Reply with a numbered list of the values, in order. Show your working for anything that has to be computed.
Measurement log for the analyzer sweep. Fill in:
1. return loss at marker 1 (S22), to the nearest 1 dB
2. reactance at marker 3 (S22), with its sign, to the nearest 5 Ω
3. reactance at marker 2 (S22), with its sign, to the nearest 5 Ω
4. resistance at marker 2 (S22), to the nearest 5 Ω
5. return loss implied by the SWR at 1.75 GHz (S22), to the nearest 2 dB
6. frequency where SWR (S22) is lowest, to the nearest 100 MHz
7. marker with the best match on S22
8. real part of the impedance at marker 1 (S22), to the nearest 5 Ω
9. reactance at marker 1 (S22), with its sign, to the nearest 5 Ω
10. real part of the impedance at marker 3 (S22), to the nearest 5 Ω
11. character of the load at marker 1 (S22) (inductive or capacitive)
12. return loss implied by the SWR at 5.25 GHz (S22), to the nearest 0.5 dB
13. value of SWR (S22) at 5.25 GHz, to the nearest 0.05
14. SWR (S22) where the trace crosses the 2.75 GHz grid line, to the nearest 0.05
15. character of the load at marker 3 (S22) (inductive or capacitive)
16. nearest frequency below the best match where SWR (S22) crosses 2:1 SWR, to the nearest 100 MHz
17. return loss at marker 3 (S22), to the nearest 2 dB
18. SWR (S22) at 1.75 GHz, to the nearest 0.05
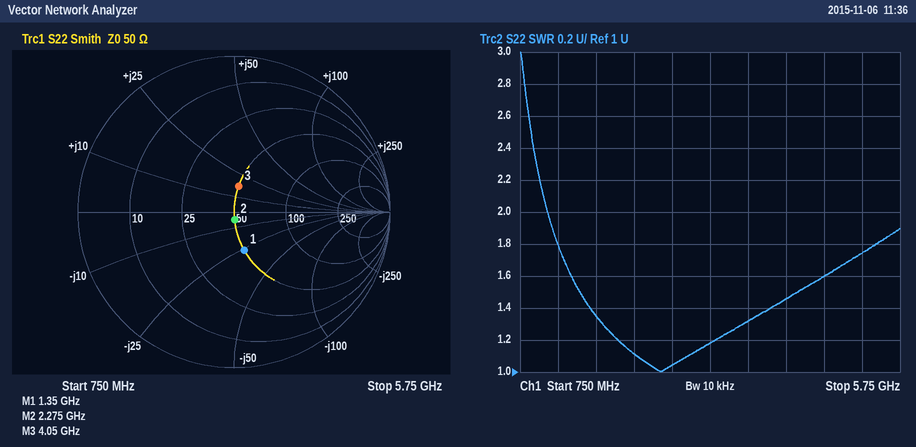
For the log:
1. 12 dB
2. +15 Ω
3. -5 Ω
4. 50 Ω
5. −20 log10((1.35 − 1)/(1.35 + 1)) ≈ 16 dB
6. 2.6 GHz
7. marker 2
8. 50 Ω
9. -25 Ω
10. 50 Ω
11. capacitive
12. −20 log10((1.75 − 1)/(1.75 + 1)) ≈ 11.3 dB, so 11.5 dB to the nearest 0.5 dB
13. 1.75
14. 1.05
15. inductive
16. 1.1 GHz
17. 16 dB
18. 1.35
